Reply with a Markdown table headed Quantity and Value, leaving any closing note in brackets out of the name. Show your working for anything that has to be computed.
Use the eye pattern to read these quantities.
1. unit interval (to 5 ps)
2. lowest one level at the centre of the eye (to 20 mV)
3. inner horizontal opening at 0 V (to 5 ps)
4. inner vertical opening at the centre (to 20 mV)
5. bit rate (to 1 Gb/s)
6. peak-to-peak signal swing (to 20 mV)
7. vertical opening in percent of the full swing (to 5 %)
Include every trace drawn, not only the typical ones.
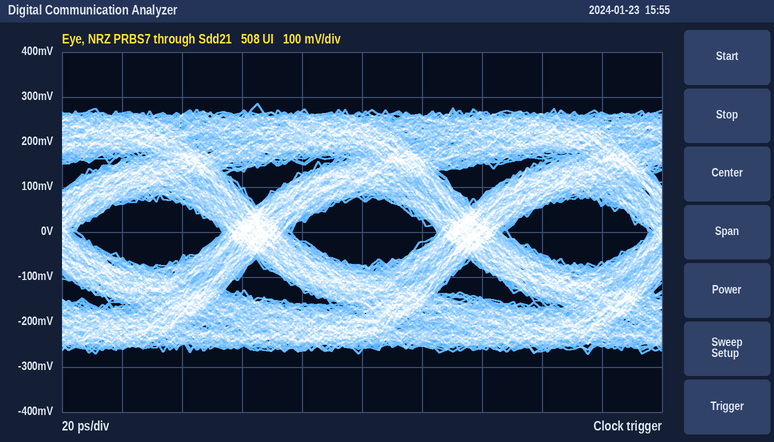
| Quantity | Value |
|---|---|
| unit interval | 70 ps |
| lowest one level at the centre of the eye | 80 mV |
| inner horizontal opening at 0 V | 50 ps |
| inner vertical opening at the centre | 140 mV |
| bit rate | 14 Gb/s |
| peak-to-peak signal swing | 560 mV |
| vertical opening in percent of the full swing | 140 mV / 560 mV ≈ 25 % |
